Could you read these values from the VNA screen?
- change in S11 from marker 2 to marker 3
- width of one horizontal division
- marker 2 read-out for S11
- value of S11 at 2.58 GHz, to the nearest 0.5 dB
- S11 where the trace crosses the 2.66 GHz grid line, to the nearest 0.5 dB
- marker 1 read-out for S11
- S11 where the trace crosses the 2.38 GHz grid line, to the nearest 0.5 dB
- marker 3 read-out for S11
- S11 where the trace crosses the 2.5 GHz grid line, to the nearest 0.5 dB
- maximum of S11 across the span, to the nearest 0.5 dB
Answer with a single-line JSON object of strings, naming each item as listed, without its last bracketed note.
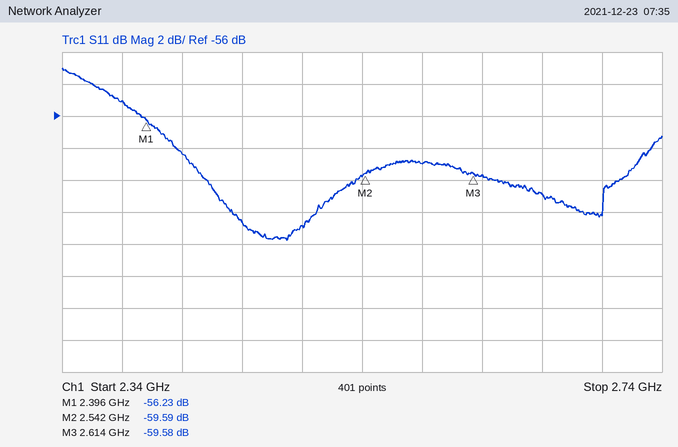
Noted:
{"change in S11 from marker 2 to marker 3": "0.01 dB", "width of one horizontal division": "40 MHz", "marker 2 read-out for S11": "-59.59 dB", "value of S11 at 2.58 GHz, to the nearest 0.5 dB": "-59.0 dB", "S11 where the trace crosses the 2.66 GHz grid line, to the nearest 0.5 dB": "-61.0 dB", "marker 1 read-out for S11": "-56.23 dB", "S11 where the trace crosses the 2.38 GHz grid line, to the nearest 0.5 dB": "-55.0 dB", "marker 3 read-out for S11": "-59.58 dB", "S11 where the trace crosses the 2.5 GHz grid line, to the nearest 0.5 dB": "-63.0 dB", "maximum of S11 across the span, to the nearest 0.5 dB": "-53.0 dB"}
